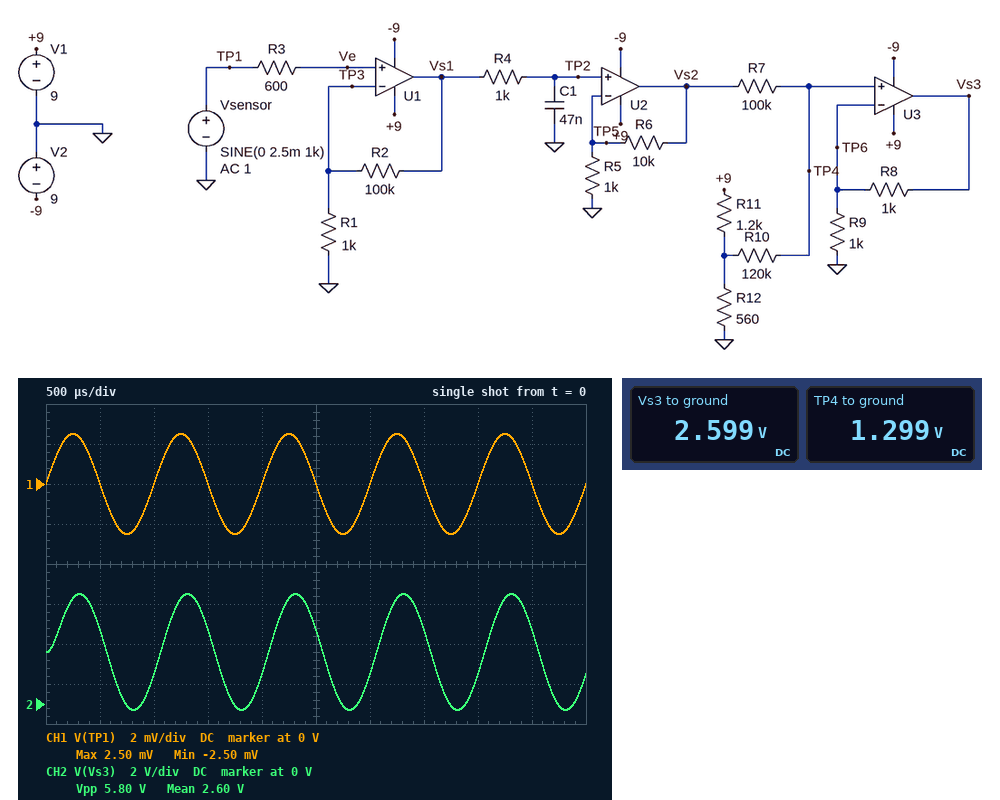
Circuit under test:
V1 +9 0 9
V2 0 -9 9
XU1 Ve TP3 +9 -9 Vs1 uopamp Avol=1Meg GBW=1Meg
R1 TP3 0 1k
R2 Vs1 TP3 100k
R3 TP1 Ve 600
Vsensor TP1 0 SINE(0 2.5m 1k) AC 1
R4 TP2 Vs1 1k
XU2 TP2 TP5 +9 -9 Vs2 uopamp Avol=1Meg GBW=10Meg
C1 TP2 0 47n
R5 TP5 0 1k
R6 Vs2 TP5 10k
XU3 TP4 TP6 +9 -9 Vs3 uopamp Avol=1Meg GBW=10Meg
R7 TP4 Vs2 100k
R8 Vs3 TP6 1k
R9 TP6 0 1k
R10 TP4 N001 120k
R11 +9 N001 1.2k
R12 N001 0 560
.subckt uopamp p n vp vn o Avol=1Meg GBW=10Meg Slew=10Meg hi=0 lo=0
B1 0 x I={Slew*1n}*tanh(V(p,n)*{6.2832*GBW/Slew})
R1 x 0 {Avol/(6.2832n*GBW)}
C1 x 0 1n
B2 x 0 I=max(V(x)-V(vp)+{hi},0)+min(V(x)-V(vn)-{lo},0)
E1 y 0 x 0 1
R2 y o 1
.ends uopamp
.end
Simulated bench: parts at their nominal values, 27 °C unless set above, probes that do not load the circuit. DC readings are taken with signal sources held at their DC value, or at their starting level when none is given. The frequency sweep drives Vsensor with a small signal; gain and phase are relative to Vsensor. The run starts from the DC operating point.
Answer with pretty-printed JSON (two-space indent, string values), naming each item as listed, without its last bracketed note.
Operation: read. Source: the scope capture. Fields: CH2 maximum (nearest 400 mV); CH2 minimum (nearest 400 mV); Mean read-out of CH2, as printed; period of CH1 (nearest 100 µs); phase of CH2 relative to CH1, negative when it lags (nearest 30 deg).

{
  "CH2 maximum": "5.6 V",
  "CH2 minimum": "-400 mV",
  "Mean read-out of CH2, as printed": "2.60 V",
  "period of CH1": "1.0 ms",
  "phase of CH2 relative to CH1, negative when it lags": "-30 deg"
}
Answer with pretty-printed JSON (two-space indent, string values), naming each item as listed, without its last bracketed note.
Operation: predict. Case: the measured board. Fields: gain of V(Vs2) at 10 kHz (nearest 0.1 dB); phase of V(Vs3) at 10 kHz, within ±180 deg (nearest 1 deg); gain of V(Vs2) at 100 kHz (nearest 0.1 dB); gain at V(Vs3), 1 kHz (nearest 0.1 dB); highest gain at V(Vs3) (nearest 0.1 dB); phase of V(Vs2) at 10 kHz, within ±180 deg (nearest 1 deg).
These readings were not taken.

{
  "gain of V(Vs2) at 10 kHz": "48.0 dB",
  "phase of V(Vs3) at 10 kHz, within ±180 deg": "-117 deg",
  "gain of V(Vs2) at 100 kHz": "11.3 dB",
  "gain at V(Vs3), 1 kHz": "61.3 dB",
  "highest gain at V(Vs3)": "61.7 dB",
  "phase of V(Vs2) at 10 kHz, within ±180 deg": "-117 deg"
}
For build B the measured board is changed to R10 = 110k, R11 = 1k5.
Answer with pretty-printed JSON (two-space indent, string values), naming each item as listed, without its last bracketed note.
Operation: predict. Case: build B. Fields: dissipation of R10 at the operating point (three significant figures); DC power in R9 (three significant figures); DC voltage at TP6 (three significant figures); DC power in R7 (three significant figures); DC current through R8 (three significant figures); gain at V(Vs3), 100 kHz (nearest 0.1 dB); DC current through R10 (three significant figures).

{
  "dissipation of R10 at the operating point": "14.9 µW",
  "DC power in R9": "1.35 mW",
  "DC voltage at TP6": "1.16 V",
  "DC power in R7": "13.5 µW",
  "DC current through R8": "1.16 mA",
  "gain at V(Vs3), 100 kHz": "11.7 dB",
  "DC current through R10": "11.6 µA"
}
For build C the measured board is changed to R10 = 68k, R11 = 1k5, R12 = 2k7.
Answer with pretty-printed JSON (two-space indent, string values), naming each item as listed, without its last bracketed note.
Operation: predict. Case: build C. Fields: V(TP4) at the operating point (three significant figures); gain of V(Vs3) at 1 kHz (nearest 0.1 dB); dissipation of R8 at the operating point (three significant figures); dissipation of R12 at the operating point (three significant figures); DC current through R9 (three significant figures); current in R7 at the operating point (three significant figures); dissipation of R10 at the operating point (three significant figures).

{
  "V(TP4) at the operating point": "3.42 V",
  "gain of V(Vs3) at 1 kHz": "58.7 dB",
  "dissipation of R8 at the operating point": "11.7 mW",
  "dissipation of R12 at the operating point": "12.3 mW",
  "DC current through R9": "3.42 mA",
  "current in R7 at the operating point": "34.2 µA",
  "dissipation of R10 at the operating point": "79.7 µW"
}
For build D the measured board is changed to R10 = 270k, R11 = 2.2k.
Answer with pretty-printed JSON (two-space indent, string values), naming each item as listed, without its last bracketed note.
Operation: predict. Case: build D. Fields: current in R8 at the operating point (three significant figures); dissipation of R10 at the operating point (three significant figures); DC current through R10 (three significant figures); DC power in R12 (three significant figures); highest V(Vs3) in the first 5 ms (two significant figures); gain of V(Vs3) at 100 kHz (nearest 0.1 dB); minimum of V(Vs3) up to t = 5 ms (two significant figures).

{
  "current in R8 at the operating point": "493 µA",
  "dissipation of R10 at the operating point": "6.56 µW",
  "DC current through R10": "4.93 µA",
  "DC power in R12": "5.94 mW",
  "highest V(Vs3) in the first 5 ms": "4.9 V",
  "gain of V(Vs3) at 100 kHz": "14.6 dB",
  "minimum of V(Vs3) up to t = 5 ms": "-2.9 V"
}
